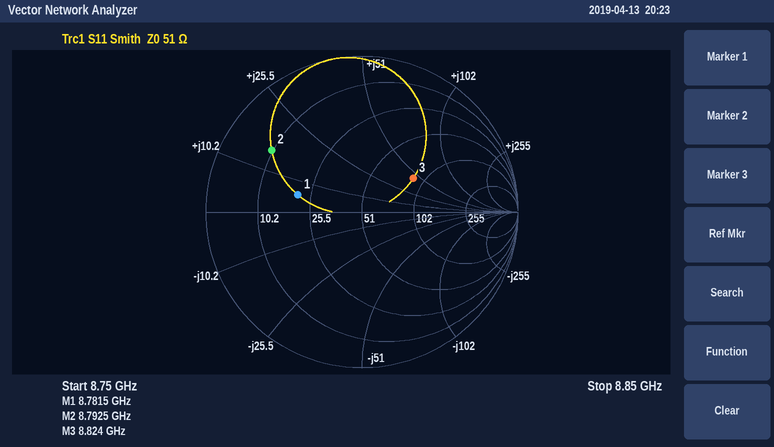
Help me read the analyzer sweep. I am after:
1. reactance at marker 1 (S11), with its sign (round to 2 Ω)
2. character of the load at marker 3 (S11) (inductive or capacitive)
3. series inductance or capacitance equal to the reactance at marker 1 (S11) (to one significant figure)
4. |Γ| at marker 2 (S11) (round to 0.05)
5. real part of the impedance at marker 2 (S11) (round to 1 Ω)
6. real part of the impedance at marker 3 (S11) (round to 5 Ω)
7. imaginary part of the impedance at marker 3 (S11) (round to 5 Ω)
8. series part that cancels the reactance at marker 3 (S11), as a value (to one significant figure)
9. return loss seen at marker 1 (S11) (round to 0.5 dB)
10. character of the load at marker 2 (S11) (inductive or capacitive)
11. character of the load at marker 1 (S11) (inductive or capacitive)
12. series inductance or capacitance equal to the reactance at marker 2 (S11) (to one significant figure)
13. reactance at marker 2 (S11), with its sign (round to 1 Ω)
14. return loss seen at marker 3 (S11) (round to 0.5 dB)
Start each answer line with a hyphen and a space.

- +6 Ω
- inductive
- 100 pH
- 0.70
- 10 Ω
- 85 Ω
- +45 Ω
- 400 fF
- 7.5 dB
- inductive
- inductive
- 300 pH
- +15 Ω
- 8.0 dB
